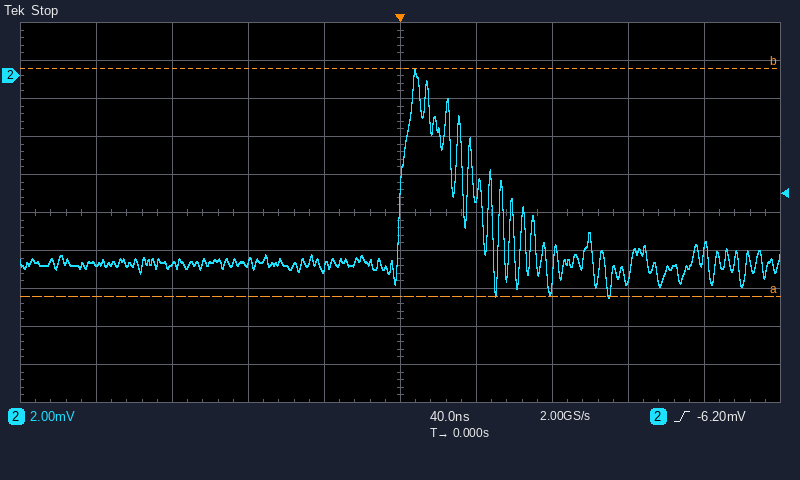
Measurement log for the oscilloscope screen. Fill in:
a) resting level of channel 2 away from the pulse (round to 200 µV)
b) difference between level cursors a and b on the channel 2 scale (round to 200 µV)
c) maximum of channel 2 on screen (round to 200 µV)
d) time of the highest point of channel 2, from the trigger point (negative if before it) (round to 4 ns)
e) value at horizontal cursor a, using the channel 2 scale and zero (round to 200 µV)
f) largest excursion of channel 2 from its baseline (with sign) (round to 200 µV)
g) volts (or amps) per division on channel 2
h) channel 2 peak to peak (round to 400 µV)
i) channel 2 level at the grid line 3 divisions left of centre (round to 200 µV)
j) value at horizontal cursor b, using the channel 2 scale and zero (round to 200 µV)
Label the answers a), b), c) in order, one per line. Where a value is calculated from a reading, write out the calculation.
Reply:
a) -9.8 mV
b) 12.0 mV
c) 400 µV
d) +8 ns
e) -11.6 mV
f) 400 µV − (-9.8 mV) = +10.2 mV
g) 2 mV
h) 12.0 mV
i) -10.0 mV
j) 400 µV
